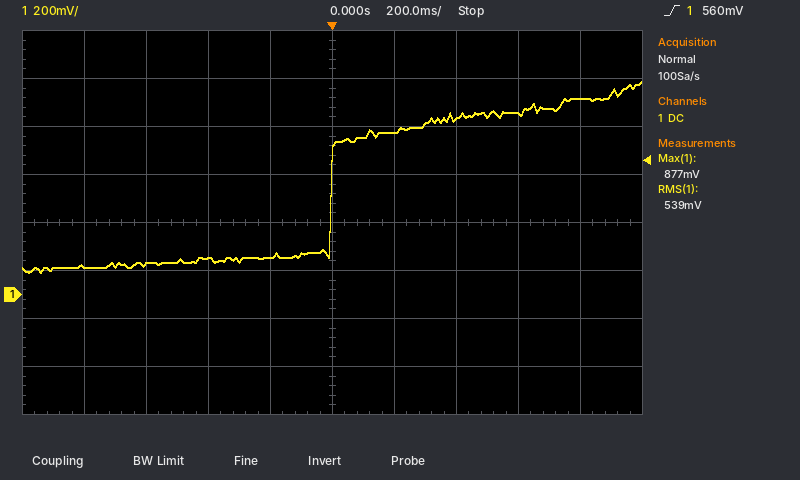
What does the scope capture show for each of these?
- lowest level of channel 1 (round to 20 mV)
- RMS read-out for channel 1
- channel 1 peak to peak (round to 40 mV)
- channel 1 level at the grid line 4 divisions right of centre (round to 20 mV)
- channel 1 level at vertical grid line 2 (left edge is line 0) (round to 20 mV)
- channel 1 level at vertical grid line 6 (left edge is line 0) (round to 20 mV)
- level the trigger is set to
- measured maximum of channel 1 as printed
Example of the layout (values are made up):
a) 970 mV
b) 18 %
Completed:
a) 100 mV
b) 539 mV
c) 800 mV
d) 820 mV
e) 120 mV
f) 680 mV
g) 560 mV
h) 877 mV
